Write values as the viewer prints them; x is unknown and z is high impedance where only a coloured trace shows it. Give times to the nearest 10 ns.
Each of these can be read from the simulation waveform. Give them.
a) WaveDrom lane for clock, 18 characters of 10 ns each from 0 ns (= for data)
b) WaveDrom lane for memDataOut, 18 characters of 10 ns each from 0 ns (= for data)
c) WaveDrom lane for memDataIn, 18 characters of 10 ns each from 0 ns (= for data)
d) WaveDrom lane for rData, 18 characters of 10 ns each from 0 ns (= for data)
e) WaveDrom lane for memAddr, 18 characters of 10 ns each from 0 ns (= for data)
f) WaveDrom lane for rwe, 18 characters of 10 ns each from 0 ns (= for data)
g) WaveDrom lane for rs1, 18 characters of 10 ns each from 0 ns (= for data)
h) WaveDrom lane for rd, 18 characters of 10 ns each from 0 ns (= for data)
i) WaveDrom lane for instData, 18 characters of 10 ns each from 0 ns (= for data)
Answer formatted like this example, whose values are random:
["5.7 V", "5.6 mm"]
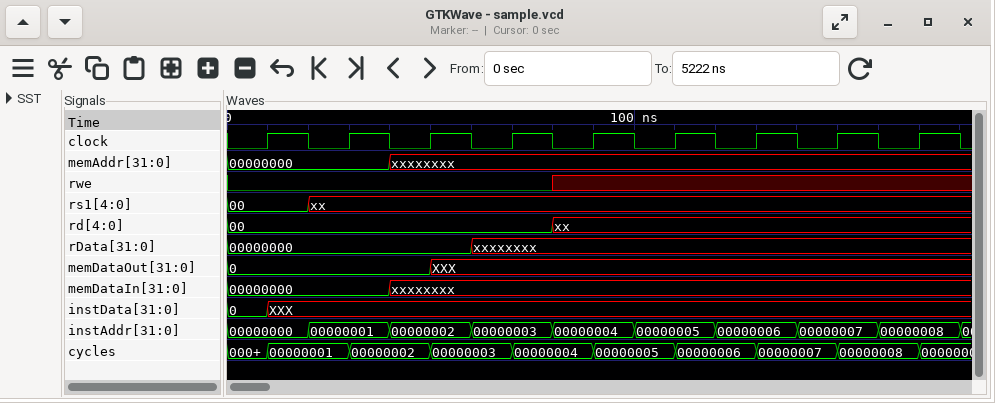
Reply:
["{name: 'clock', wave: '010101010101010101'}", "{name: 'memDataOut', wave: '=....x............', data: '0'}", "{name: 'memDataIn', wave: '=...x.............', data: '00000000'}", "{name: 'rData', wave: '=.....x...........', data: '00000000'}", "{name: 'memAddr', wave: '=...x.............', data: '00000000'}", "{name: 'rwe', wave: '0.......x.........'}", "{name: 'rs1', wave: '=.x...............', data: '00'}", "{name: 'rd', wave: '=.......x.........', data: '00'}", "{name: 'instData', wave: '=x................', data: '0'}"]
